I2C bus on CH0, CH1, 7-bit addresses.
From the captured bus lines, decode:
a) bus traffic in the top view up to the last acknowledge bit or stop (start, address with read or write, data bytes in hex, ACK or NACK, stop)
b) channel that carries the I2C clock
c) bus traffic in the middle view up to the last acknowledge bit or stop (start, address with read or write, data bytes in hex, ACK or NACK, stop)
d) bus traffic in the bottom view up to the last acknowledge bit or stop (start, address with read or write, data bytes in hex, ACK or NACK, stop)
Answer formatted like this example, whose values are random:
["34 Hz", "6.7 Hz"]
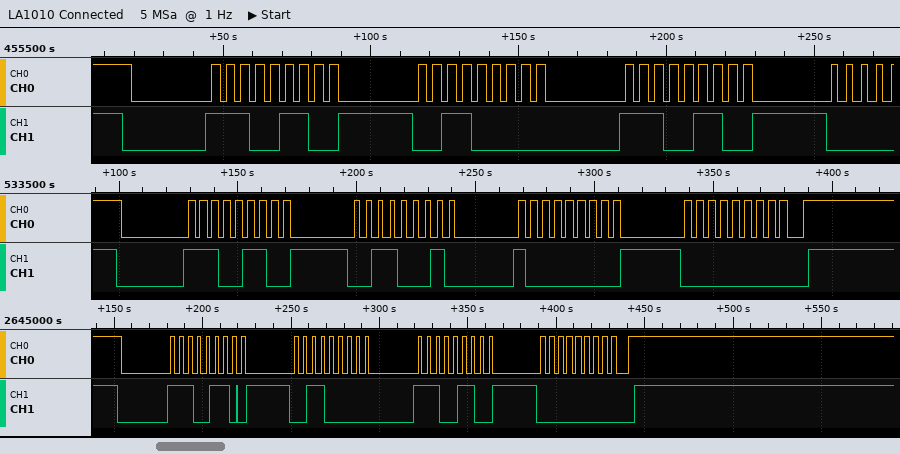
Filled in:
["start, address 73 write ACK, 30 ACK, E6 ACK", "CH0", "start, address 73 write ACK, 31 ACK, 80 ACK, 00 ACK, stop", "start, address 73 write ACK, 30 ACK, E6 ACK, 00 ACK, stop"]
